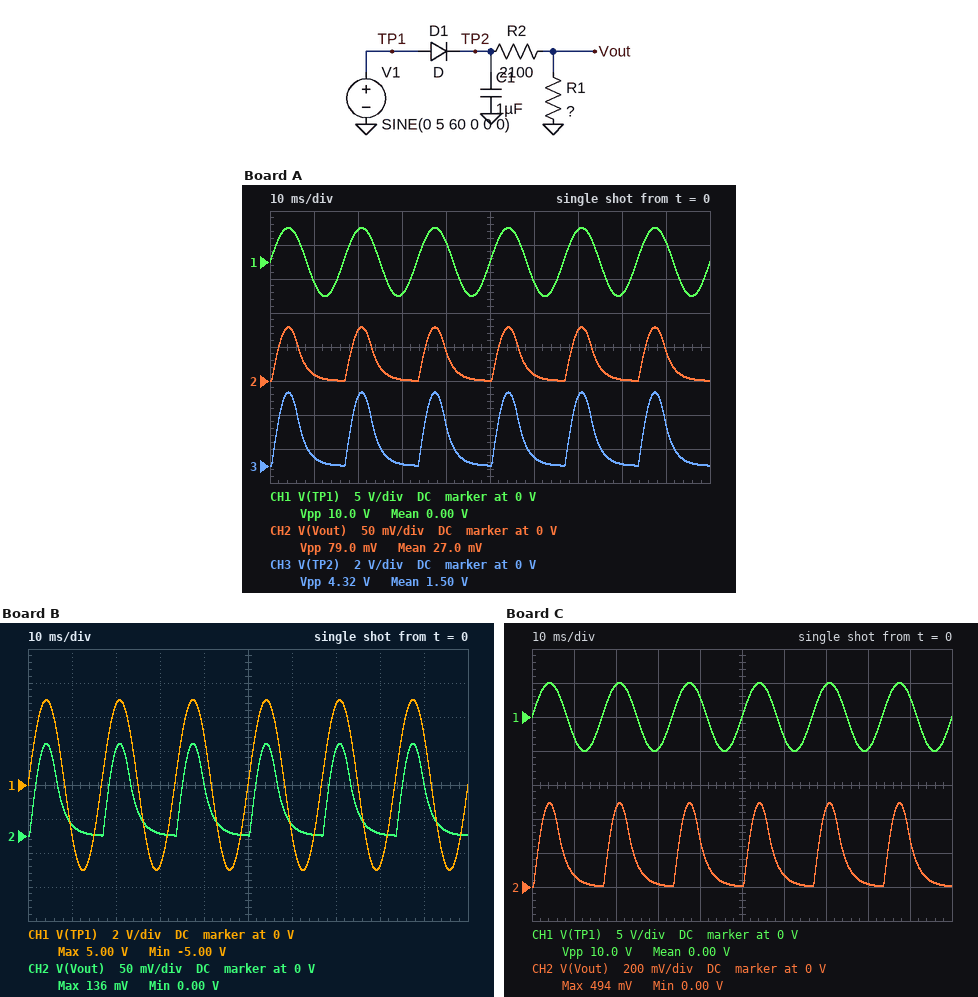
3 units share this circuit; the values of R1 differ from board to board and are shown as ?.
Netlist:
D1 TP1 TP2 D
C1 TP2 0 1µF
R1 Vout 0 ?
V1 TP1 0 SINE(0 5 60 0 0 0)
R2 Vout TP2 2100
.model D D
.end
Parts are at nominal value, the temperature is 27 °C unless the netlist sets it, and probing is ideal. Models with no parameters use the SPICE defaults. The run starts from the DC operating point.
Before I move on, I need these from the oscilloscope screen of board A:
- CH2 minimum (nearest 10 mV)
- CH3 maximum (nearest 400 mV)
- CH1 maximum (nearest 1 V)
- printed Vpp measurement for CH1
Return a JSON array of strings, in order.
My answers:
["0 V", "4.4 V", "5 V", "10.0 V"]
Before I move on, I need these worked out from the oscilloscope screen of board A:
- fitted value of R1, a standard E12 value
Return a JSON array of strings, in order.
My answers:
["39 Ω"]
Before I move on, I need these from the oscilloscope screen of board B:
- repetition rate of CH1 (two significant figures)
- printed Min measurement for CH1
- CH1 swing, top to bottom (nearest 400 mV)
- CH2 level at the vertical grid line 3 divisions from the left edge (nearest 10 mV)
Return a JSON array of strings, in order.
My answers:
["60 Hz", "-5.00 V", "10.0 V", "0 V"]
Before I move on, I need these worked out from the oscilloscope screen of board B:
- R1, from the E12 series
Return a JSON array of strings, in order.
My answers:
["68 Ω"]
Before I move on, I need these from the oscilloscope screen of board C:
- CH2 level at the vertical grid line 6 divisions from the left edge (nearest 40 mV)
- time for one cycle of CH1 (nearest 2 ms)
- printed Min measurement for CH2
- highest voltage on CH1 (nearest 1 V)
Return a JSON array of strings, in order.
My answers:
["80 mV", "16 ms", "0.00 V", "5 V"]
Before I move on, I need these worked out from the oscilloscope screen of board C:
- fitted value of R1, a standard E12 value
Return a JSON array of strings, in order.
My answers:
["270 Ω"]
